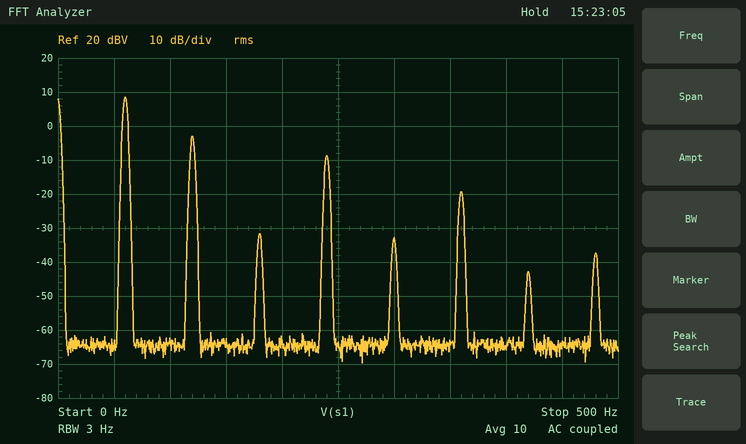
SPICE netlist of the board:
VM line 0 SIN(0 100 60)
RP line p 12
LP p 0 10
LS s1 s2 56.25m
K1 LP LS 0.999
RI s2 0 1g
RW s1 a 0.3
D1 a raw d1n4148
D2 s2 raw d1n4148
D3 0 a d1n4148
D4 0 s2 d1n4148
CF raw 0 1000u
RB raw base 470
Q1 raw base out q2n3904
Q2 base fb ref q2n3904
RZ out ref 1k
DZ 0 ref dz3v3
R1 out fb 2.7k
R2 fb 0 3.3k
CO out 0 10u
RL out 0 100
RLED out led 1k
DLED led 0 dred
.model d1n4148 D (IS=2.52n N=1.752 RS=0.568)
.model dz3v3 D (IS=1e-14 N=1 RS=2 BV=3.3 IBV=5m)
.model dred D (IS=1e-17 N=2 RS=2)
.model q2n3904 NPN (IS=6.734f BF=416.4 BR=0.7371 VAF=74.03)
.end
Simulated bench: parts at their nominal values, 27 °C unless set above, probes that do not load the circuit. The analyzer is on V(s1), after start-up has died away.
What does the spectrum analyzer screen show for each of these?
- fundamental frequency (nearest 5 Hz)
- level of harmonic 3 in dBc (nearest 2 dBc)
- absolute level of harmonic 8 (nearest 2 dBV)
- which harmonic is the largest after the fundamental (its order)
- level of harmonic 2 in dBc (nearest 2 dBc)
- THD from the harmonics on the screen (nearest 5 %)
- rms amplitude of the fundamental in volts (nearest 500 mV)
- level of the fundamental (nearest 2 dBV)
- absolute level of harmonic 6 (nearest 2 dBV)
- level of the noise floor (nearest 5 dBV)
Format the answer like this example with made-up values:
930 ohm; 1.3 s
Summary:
60 Hz; -40 dBc; -38 dBV; 2; -12 dBc; 30 %; 2.5 V; 8 dBV; -20 dBV; -65 dBV
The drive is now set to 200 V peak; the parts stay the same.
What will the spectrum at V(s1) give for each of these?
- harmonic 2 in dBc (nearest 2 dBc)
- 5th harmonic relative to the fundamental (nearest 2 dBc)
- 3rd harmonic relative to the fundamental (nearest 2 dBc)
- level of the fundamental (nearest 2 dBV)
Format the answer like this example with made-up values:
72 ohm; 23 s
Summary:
-10 dBc; -48 dBc; -44 dBc; 14 dBV
